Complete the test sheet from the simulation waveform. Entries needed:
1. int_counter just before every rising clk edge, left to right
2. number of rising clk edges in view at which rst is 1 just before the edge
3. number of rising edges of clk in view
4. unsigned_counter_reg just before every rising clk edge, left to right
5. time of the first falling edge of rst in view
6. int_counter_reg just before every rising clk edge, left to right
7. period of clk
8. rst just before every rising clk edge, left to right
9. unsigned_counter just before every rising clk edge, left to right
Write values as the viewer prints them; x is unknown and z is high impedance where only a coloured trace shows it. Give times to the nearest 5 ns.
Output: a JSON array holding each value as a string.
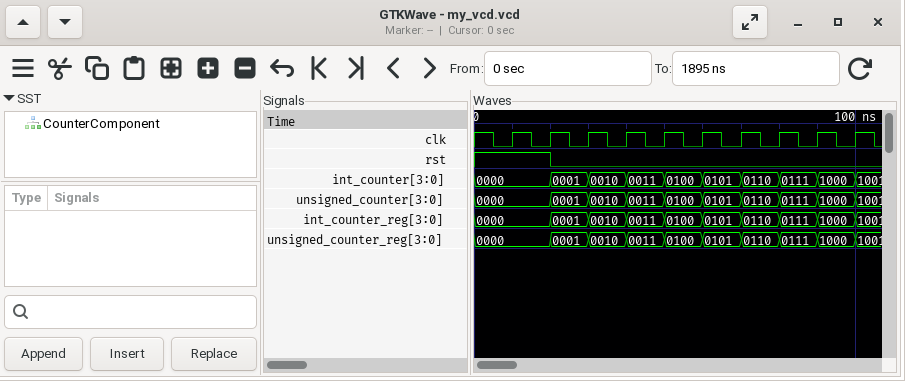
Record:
["0000, 0000, 0001, 0010, 0011, 0100, 0101, 0110, 0111, 1000", "2", "10", "0000, 0000, 0001, 0010, 0011, 0100, 0101, 0110, 0111, 1000", "20 ns", "0000, 0000, 0001, 0010, 0011, 0100, 0101, 0110, 0111, 1000", "10 ns", "1 1 0 0 0 0 0 0 0 0", "0000, 0000, 0001, 0010, 0011, 0100, 0101, 0110, 0111, 1000"]
